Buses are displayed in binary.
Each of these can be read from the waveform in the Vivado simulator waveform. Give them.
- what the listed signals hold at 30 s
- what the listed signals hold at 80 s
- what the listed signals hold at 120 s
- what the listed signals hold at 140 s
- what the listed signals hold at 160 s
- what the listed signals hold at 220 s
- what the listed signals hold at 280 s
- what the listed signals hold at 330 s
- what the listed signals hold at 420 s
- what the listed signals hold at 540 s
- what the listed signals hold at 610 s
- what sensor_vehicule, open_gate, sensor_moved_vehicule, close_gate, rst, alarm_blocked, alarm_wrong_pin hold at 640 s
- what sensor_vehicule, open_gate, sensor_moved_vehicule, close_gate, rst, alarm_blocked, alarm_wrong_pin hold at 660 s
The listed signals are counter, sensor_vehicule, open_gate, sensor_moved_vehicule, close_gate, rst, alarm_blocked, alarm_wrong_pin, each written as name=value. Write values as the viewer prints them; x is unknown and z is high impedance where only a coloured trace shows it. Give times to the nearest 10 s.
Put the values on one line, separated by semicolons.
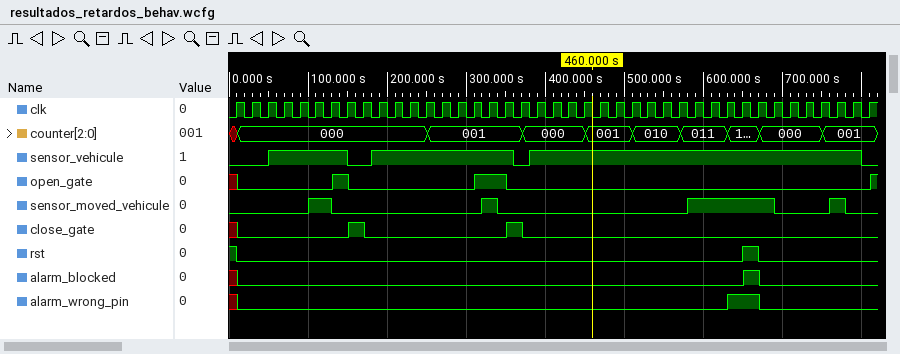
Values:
counter=000, sensor_vehicule=0, open_gate=0, sensor_moved_vehicule=0, close_gate=0, rst=0, alarm_blocked=0, alarm_wrong_pin=0; counter=000, sensor_vehicule=1, open_gate=0, sensor_moved_vehicule=0, close_gate=0, rst=0, alarm_blocked=0, alarm_wrong_pin=0; counter=000, sensor_vehicule=1, open_gate=0, sensor_moved_vehicule=1, close_gate=0, rst=0, alarm_blocked=0, alarm_wrong_pin=0; counter=000, sensor_vehicule=1, open_gate=1, sensor_moved_vehicule=0, close_gate=0, rst=0, alarm_blocked=0, alarm_wrong_pin=0; counter=000, sensor_vehicule=0, open_gate=0, sensor_moved_vehicule=0, close_gate=1, rst=0, alarm_blocked=0, alarm_wrong_pin=0; counter=000, sensor_vehicule=1, open_gate=0, sensor_moved_vehicule=0, close_gate=0, rst=0, alarm_blocked=0, alarm_wrong_pin=0; counter=001, sensor_vehicule=1, open_gate=0, sensor_moved_vehicule=0, close_gate=0, rst=0, alarm_blocked=0, alarm_wrong_pin=0; counter=001, sensor_vehicule=1, open_gate=1, sensor_moved_vehicule=1, close_gate=0, rst=0, alarm_blocked=0, alarm_wrong_pin=0; counter=000, sensor_vehicule=1, open_gate=0, sensor_moved_vehicule=0, close_gate=0, rst=0, alarm_blocked=0, alarm_wrong_pin=0; counter=010, sensor_vehicule=1, open_gate=0, sensor_moved_vehicule=0, close_gate=0, rst=0, alarm_blocked=0, alarm_wrong_pin=0; counter=011, sensor_vehicule=1, open_gate=0, sensor_moved_vehicule=1, close_gate=0, rst=0, alarm_blocked=0, alarm_wrong_pin=0; sensor_vehicule=1, open_gate=0, sensor_moved_vehicule=1, close_gate=0, rst=0, alarm_blocked=0, alarm_wrong_pin=1; sensor_vehicule=1, open_gate=0, sensor_moved_vehicule=1, close_gate=0, rst=1, alarm_blocked=1, alarm_wrong_pin=1
